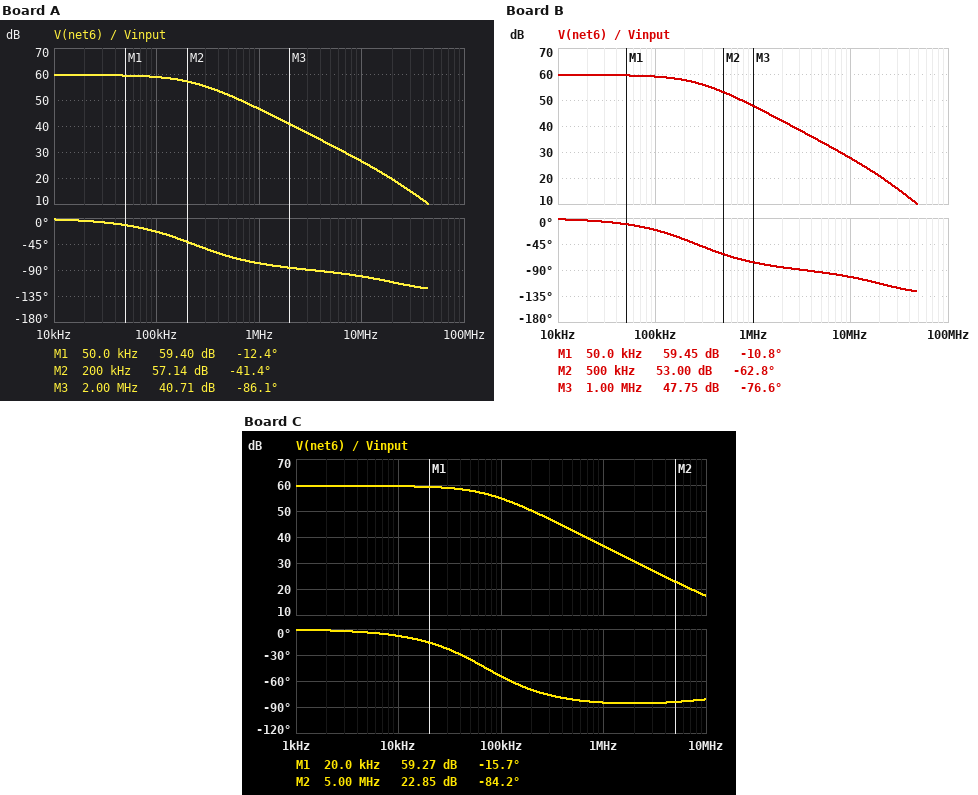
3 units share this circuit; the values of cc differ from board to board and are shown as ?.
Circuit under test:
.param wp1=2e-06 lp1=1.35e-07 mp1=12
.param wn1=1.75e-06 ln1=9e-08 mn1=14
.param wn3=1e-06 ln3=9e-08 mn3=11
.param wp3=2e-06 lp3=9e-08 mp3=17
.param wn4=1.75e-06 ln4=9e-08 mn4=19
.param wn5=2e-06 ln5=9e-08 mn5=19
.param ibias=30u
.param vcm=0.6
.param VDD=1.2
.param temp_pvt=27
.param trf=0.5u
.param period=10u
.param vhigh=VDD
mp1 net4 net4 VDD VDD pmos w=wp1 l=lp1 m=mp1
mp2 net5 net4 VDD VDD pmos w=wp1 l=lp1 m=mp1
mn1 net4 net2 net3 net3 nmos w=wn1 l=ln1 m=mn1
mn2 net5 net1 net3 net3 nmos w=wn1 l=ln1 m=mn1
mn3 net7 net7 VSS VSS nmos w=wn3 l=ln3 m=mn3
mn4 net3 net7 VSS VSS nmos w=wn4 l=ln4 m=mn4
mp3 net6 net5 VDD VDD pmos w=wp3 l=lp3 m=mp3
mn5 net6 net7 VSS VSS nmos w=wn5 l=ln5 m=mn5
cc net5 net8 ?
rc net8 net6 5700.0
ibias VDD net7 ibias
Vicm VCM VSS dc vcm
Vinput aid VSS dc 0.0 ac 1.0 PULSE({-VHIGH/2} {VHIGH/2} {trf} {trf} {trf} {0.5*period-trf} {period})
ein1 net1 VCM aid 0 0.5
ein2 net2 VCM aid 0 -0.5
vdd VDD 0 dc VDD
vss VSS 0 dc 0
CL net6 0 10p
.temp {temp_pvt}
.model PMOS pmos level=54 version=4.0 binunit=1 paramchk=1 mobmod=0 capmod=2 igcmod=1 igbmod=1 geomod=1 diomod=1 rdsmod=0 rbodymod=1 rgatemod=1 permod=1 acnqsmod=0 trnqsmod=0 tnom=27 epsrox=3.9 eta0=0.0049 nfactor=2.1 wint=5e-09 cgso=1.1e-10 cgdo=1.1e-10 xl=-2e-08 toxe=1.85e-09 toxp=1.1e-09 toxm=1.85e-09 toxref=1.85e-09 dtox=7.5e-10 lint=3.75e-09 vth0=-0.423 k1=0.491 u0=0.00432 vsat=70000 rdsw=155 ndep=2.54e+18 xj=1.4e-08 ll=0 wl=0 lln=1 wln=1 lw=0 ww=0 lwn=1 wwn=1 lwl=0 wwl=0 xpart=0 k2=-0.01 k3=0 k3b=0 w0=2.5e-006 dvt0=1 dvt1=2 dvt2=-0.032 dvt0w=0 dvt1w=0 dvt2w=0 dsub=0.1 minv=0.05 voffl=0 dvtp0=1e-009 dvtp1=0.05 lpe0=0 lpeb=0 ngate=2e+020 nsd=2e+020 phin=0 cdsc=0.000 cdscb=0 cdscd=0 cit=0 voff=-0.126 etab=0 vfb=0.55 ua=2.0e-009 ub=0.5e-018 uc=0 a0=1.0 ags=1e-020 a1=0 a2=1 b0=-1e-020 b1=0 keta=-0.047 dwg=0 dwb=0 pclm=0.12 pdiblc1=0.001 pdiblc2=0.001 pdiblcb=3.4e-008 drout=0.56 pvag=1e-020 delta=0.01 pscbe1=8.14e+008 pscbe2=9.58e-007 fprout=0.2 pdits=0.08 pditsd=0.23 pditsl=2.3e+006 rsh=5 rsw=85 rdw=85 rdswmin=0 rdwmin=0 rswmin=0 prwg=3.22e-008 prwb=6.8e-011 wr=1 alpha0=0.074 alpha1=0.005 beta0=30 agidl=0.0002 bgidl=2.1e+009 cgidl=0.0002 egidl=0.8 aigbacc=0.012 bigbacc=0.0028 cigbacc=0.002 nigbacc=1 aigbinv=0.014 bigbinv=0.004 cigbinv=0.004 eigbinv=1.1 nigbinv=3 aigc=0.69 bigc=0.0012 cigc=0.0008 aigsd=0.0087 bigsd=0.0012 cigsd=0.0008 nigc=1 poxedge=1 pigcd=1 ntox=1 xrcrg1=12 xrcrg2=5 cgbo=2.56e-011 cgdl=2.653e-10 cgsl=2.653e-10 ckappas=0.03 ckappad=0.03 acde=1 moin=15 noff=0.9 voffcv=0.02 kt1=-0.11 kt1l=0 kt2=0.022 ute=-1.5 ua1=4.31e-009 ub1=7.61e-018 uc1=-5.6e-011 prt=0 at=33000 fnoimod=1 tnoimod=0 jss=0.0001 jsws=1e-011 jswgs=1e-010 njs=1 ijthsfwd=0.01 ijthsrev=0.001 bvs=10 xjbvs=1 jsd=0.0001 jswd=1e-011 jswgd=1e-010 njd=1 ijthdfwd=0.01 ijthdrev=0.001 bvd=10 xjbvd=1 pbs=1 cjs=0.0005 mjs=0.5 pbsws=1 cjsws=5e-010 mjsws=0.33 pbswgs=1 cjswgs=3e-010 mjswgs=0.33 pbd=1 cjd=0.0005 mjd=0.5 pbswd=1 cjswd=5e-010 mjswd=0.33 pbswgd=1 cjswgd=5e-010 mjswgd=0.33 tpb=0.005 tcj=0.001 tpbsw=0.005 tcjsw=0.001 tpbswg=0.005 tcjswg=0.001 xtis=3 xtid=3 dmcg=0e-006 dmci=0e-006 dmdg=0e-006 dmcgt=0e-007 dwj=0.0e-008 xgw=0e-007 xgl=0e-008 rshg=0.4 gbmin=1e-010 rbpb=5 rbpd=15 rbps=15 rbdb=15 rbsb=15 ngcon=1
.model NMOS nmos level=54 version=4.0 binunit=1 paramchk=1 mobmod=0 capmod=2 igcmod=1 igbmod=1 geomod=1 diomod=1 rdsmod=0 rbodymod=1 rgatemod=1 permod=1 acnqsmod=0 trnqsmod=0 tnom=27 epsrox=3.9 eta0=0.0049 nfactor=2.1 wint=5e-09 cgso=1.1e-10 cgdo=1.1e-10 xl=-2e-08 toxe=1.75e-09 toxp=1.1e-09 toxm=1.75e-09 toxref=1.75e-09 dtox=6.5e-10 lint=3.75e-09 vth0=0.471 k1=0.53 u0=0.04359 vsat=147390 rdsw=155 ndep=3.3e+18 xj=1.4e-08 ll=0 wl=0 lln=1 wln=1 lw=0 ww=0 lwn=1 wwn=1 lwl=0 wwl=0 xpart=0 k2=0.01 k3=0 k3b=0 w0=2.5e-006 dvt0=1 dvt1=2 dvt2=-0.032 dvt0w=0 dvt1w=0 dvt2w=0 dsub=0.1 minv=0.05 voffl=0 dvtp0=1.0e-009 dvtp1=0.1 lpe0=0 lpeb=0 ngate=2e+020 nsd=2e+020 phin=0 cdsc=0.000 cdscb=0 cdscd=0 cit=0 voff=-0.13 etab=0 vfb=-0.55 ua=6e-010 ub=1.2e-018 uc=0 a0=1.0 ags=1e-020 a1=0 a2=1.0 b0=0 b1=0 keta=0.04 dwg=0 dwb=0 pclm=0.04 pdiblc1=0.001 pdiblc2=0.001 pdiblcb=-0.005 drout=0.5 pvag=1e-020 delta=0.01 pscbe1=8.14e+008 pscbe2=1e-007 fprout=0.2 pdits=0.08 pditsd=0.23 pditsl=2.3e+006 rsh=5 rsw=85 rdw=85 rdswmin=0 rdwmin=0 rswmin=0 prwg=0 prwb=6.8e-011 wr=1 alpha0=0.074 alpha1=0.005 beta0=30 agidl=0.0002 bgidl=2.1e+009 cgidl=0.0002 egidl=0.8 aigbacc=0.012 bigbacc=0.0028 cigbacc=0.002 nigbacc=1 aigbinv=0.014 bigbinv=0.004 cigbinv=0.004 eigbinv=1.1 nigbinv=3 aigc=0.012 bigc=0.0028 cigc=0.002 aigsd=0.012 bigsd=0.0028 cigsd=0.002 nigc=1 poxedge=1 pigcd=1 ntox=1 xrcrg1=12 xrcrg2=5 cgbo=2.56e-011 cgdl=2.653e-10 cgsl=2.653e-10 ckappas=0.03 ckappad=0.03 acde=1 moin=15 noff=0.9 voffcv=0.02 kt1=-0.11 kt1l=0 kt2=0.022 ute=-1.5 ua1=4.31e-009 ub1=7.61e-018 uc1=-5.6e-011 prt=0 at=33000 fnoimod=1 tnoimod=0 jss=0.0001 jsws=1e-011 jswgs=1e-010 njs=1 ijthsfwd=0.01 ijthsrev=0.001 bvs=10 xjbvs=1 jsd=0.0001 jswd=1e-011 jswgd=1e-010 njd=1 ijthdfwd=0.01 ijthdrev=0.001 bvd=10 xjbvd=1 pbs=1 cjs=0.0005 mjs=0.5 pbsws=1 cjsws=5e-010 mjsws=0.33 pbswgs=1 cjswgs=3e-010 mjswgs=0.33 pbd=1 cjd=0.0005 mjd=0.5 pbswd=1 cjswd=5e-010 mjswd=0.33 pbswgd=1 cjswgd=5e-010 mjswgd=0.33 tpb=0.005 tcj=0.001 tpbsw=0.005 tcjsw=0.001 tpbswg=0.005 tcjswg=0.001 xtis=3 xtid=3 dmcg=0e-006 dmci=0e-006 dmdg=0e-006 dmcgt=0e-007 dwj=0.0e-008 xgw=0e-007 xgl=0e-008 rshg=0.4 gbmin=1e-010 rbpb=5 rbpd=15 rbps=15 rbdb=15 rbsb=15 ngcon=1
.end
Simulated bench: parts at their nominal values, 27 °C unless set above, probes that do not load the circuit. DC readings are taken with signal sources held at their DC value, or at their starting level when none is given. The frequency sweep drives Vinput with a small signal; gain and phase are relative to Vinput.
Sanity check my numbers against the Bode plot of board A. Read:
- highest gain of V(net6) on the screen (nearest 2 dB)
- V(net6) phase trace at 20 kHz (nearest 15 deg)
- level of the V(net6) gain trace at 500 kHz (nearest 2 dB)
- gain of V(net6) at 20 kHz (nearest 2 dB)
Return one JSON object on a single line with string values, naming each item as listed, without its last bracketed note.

{"highest gain of V(net6) on the screen": "60 dB", "V(net6) phase trace at 20 kHz": "0 deg", "level of the V(net6) gain trace at 500 kHz": "52 dB", "gain of V(net6) at 20 kHz": "60 dB"}
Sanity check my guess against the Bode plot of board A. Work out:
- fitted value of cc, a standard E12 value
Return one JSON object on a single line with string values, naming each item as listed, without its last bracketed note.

{"fitted value of cc, a standard E12 value": "470 fF"}
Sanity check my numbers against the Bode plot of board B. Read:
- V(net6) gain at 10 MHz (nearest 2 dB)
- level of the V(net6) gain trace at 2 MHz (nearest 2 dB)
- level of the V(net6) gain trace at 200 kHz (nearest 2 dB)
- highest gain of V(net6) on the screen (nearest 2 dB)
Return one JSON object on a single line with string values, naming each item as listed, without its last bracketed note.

{"V(net6) gain at 10 MHz": "28 dB", "level of the V(net6) gain trace at 2 MHz": "42 dB", "level of the V(net6) gain trace at 200 kHz": "58 dB", "highest gain of V(net6) on the screen": "60 dB"}
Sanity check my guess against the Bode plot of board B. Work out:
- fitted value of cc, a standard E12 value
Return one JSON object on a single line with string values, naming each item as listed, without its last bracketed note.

{"fitted value of cc, a standard E12 value": "390 fF"}
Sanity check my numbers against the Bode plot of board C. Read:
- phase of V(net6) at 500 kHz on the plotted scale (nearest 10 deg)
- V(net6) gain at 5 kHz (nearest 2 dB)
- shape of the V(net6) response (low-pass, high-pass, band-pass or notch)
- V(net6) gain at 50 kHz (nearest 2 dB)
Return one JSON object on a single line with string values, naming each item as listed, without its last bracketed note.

{"phase of V(net6) at 500 kHz on the plotted scale": "-80 deg", "V(net6) gain at 5 kHz": "60 dB", "shape of the V(net6) response": "low-pass", "V(net6) gain at 50 kHz": "58 dB"}
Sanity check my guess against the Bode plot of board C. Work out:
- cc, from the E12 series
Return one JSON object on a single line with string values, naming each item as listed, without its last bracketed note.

{"cc, from the E12 series": "1.8 pF"}
